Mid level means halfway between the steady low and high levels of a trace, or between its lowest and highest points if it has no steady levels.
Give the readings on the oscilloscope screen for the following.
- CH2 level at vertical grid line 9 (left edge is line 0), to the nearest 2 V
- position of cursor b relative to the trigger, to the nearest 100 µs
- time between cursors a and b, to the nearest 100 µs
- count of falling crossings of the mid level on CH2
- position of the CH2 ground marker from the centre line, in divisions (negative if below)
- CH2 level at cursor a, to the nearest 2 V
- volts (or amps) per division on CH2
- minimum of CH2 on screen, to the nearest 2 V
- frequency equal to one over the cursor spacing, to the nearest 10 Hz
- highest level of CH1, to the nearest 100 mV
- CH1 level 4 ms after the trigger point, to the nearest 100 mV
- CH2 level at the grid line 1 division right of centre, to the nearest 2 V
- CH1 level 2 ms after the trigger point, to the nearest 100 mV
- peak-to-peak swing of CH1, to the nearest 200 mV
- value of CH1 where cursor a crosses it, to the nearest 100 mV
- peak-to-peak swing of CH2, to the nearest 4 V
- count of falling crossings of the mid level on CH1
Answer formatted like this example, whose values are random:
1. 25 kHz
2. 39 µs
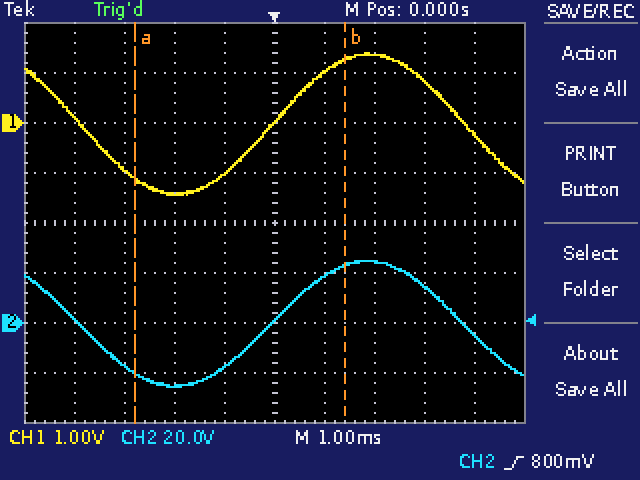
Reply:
1. -4 V
2. +1.4 ms
3. 4.2 ms
4. 2
5. -2.0 div
6. -20 V
7. 20 V
8. -26 V
9. 240 Hz
10. 1.4 V
11. -200 mV
12. 18 V
13. 1.4 V
14. 2.8 V
15. -1.1 V
16. 52 V
17. 2
